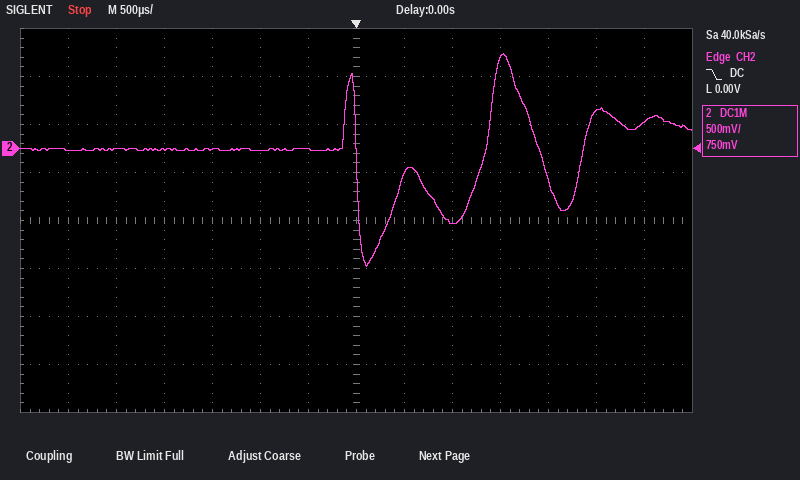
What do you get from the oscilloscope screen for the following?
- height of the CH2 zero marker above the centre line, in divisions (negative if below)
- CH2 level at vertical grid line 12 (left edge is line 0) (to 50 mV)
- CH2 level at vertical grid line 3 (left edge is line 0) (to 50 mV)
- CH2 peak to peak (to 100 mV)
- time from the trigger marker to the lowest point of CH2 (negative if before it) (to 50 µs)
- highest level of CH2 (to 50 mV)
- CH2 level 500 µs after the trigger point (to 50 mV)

+1.5 div
400 mV
0 mV
2.20 V
+100 µs
1.00 V
-250 mV
